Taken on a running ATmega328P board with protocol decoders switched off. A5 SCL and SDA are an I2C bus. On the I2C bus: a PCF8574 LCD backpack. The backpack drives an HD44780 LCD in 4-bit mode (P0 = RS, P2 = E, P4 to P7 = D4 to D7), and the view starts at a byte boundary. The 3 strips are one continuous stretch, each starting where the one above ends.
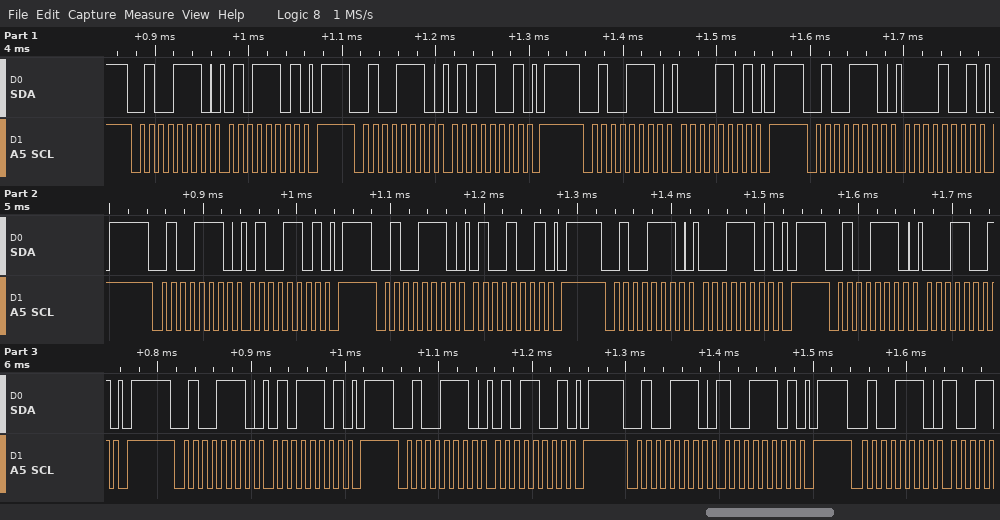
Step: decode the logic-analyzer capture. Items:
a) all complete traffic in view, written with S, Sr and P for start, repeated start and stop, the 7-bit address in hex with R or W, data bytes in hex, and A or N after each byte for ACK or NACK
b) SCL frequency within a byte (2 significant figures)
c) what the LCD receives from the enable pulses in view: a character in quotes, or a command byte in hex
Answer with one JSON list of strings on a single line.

["S 27W A 5D A P S 27W A 59 A P S 27W A 0D A P S 27W A 09 A P S 27W A 4D A P S 27W A 49 A P S 27W A 1D A P S 27W A 19 A P S 27W A 5D A P S 27W A 59 A P S 27W A 9D A P S 27W A", "100 kHz", "'P' 'A'"]
